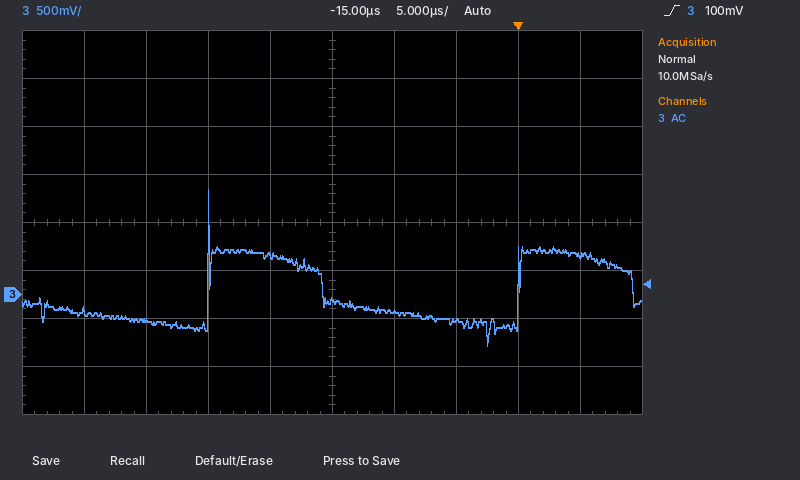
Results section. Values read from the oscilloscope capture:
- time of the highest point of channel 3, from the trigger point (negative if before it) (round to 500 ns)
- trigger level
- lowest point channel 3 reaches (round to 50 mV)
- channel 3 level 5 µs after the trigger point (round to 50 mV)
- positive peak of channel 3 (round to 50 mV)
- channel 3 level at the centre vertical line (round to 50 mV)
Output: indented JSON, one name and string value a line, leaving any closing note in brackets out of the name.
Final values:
{
  "time of the highest point of channel 3, from the trigger point (negative if before it)": "-25.0 µs",
  "trigger level": "100 mV",
  "lowest point channel 3 reaches": "-550 mV",
  "channel 3 level 5 µs after the trigger point": "400 mV",
  "positive peak of channel 3": "1.10 V",
  "channel 3 level at the centre vertical line": "-50 mV"
}
